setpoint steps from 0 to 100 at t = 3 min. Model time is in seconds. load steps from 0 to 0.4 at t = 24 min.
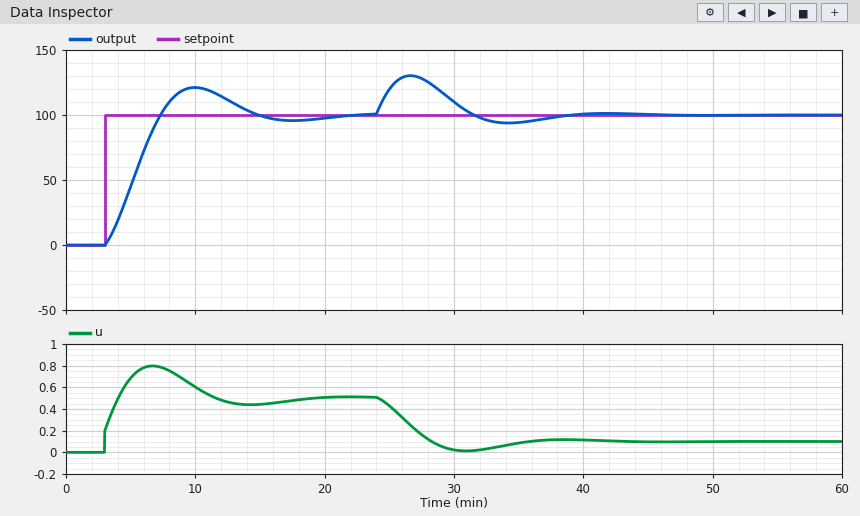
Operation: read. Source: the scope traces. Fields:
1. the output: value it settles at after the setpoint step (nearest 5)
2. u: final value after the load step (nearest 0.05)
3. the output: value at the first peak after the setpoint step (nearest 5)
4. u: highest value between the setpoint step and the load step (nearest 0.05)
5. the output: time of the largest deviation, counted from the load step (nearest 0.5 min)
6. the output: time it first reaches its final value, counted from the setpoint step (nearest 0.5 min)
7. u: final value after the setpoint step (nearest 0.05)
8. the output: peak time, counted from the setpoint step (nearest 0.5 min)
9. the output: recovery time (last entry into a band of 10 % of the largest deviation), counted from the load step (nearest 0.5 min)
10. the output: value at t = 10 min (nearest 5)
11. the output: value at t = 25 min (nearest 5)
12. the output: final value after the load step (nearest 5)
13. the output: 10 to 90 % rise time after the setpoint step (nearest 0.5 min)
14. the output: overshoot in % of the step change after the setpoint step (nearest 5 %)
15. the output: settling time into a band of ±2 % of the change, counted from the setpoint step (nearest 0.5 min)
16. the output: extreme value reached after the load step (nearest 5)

100
0.10
120
0.80
2.5 min
4.5 min
0.50
7.0 min
13.0 min
120
120
100
3.0 min
20 %
17.5 min
130
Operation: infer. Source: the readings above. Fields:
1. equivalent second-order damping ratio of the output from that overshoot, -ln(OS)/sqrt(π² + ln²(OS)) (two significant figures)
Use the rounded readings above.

0.46
